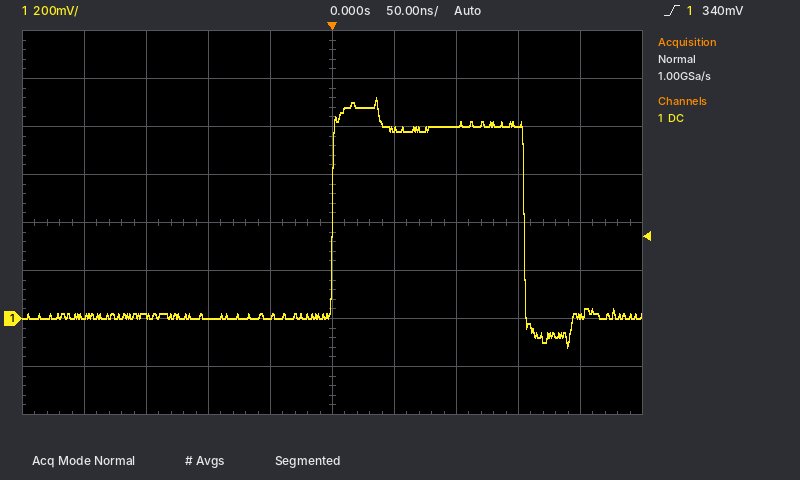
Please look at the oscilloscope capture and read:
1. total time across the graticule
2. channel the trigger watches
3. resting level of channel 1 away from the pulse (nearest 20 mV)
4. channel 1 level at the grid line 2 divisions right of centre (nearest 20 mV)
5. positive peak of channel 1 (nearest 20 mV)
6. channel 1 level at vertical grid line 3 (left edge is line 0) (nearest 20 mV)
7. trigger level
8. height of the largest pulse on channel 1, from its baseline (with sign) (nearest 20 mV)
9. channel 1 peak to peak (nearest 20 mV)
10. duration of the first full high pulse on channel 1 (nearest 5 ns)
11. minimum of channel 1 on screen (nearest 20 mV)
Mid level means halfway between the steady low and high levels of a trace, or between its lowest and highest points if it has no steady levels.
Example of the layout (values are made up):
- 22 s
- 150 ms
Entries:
- 500 ns
- channel 1
- 0 mV
- 800 mV
- 920 mV
- 0 mV
- 340 mV
- +920 mV
- 1.04 V
- 155 ns
- -120 mV
